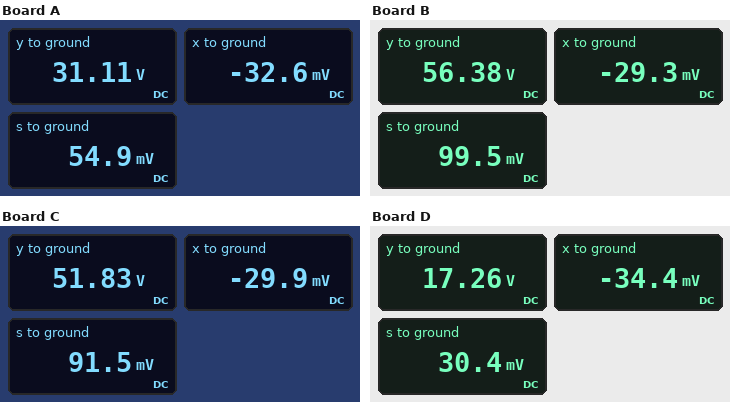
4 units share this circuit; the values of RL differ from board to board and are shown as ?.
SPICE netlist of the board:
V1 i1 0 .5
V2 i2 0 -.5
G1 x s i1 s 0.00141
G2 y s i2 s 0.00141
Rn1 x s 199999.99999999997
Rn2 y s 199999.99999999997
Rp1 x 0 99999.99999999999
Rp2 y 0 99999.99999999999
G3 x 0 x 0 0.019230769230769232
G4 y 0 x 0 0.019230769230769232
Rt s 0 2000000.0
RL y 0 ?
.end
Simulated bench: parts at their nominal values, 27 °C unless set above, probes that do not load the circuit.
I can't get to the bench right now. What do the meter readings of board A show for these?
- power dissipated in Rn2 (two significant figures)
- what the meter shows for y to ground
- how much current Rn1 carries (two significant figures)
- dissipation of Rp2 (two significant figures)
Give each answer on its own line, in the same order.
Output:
4.8 mW
31.11 V
440 nA
9.7 mW
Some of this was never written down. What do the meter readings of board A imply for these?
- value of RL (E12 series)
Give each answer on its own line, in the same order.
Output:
33 kΩ
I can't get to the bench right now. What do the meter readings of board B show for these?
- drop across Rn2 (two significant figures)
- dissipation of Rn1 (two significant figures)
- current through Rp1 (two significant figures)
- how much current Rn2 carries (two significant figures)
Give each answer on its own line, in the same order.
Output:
56 V
83 nW
290 nA
280 µA
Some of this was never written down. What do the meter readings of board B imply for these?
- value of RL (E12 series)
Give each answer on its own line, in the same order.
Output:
100 kΩ
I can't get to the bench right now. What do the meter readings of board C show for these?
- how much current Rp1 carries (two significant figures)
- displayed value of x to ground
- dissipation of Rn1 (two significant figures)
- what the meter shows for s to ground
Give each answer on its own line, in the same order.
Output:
300 nA
-29.9 mV
74 nW
91.5 mV
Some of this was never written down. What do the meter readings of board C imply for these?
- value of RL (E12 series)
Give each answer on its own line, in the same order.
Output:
82 kΩ
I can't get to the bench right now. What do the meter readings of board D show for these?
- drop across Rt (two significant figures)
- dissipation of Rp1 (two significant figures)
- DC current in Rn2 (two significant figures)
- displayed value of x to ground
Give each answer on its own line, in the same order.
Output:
30 mV
12 nW
86 µA
-34.4 mV
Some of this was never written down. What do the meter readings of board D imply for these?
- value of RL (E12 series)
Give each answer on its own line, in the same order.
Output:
15 kΩ
